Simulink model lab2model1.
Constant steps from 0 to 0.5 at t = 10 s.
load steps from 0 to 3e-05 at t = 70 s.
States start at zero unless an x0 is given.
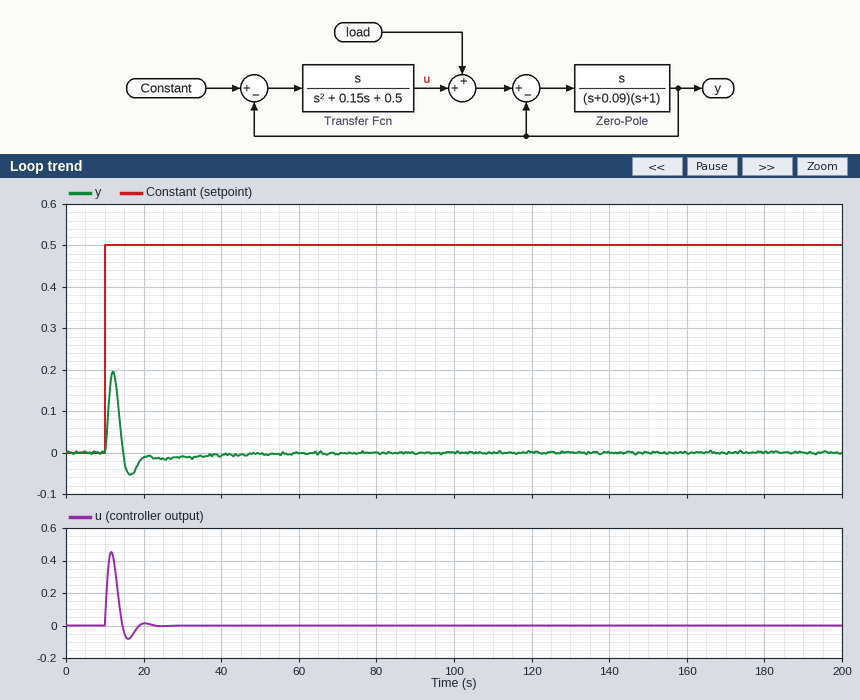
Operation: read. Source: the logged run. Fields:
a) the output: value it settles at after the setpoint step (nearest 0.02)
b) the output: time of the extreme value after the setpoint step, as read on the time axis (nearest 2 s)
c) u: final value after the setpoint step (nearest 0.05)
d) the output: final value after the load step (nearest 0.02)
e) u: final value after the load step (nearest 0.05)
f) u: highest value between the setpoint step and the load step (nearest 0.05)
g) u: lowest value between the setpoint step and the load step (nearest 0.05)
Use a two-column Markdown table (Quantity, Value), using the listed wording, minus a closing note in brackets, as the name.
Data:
| Quantity | Value |
|---|---|
| the output: value it settles at after the setpoint step | 0.00 |
| the output: time of the extreme value after the setpoint step, as read on the time axis | 12 s |
| u: final value after the setpoint step | 0.00 |
| the output: final value after the load step | 0.00 |
| u: final value after the load step | 0.00 |
| u: highest value between the setpoint step and the load step | 0.45 |
| u: lowest value between the setpoint step and the load step | -0.10 |
